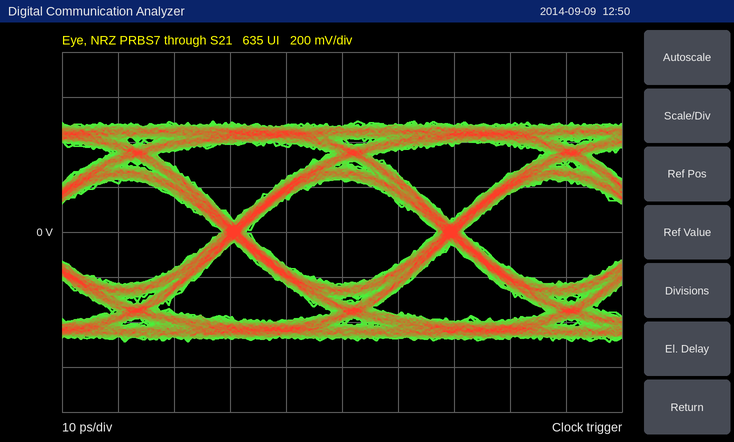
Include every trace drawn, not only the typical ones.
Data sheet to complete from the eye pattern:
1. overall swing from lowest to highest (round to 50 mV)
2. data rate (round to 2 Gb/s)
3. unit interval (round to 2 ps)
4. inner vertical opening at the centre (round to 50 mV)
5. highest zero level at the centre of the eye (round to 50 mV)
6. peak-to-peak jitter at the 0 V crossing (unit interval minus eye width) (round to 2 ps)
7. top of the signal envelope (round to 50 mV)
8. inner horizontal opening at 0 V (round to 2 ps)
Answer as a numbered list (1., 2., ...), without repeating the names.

1. 1.00 V
2. 26 Gb/s
3. 38 ps
4. 450 mV
5. -250 mV
6. 4 ps
7. 500 mV
8. 34 ps
